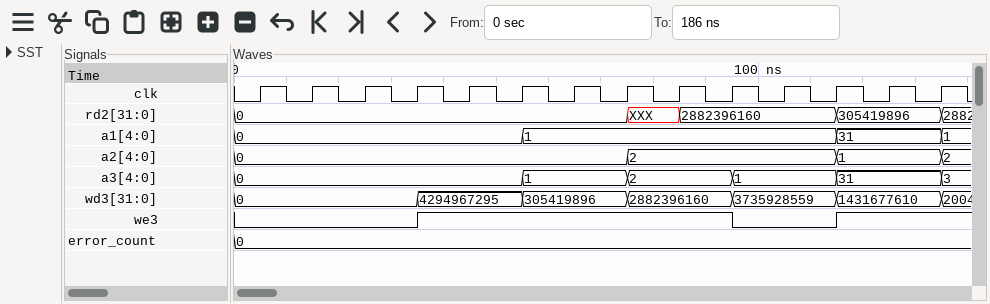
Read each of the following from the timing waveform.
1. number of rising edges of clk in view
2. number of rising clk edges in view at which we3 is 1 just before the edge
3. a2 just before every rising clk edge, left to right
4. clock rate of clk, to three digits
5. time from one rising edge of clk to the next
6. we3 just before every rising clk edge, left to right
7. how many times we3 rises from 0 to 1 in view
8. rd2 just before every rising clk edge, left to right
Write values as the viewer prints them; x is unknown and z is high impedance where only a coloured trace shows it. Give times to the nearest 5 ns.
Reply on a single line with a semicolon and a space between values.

14; 8; 0, 0, 0, 0, 0, 0, 0, 0, 2, 2, 2, 2, 1, 1; 100 MHz; 10 ns; 0 0 0 0 1 1 1 1 1 1 0 0 1 1; 2; 0, 0, 0, 0, 0, 0, 0, 0, XXX, 2882396160, 2882396160, 2882396160, 305419896, 305419896
